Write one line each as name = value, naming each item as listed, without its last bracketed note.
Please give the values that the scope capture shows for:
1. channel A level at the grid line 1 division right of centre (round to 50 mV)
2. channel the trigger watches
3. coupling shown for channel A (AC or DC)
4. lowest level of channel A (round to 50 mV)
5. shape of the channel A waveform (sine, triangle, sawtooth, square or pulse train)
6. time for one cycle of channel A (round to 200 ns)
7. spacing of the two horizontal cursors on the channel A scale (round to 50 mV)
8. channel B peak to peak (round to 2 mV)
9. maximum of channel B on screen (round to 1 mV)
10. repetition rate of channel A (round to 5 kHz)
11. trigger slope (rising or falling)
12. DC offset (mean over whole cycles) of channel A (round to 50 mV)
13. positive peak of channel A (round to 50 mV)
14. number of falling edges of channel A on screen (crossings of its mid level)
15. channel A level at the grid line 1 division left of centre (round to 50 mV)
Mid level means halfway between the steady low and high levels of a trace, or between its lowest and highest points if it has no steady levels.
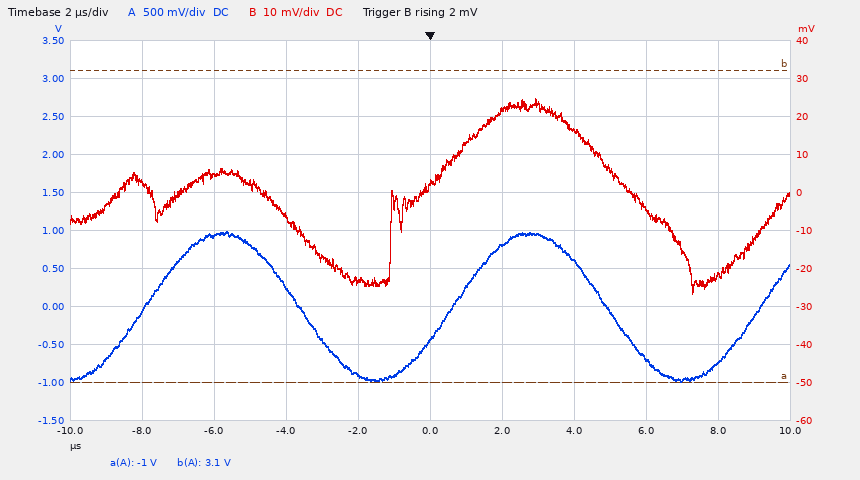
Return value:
channel A level at the grid line 1 division right of centre = 800 mV
channel the trigger watches = channel B
coupling shown for channel A = DC
lowest level of channel A = -1.00 V
shape of the channel A waveform = sine
time for one cycle of channel A = 8.6 µs
spacing of the two horizontal cursors on the channel A scale = 4.10 V
channel B peak to peak = 52 mV
maximum of channel B on screen = 25 mV
repetition rate of channel A = 115 kHz
trigger slope = rising
DC offset (mean over whole cycles) of channel A = 0 mV
positive peak of channel A = 1.00 V
number of falling edges of channel A on screen = 2
channel A level at the grid line 1 division left of centre = -900 mV
